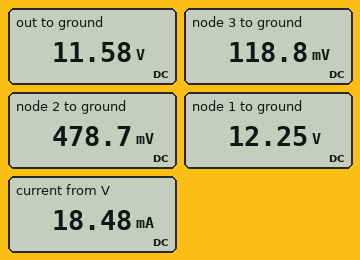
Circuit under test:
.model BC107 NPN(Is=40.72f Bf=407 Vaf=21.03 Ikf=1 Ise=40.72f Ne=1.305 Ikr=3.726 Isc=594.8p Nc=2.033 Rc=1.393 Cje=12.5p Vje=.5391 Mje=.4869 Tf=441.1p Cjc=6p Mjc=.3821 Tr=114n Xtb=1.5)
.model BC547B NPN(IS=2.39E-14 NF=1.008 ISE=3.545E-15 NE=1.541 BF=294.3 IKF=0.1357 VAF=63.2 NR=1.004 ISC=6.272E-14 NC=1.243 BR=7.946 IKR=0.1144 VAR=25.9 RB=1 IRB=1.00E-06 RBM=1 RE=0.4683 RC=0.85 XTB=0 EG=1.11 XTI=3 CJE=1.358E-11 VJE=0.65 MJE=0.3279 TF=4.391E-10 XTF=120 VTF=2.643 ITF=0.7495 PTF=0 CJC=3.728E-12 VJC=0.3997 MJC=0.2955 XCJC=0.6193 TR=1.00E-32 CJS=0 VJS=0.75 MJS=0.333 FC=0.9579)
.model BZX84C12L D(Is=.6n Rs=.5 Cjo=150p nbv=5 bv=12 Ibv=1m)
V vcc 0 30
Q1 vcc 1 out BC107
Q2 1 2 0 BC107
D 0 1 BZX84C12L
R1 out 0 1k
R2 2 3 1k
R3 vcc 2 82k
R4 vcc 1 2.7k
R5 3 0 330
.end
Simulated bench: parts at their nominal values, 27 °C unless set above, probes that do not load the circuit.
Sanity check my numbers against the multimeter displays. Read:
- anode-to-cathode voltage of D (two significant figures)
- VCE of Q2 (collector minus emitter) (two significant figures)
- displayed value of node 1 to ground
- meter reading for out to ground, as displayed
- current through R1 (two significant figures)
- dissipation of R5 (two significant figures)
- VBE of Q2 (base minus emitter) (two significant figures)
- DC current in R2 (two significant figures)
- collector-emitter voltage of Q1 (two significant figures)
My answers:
-12 V
12 V
12.25 V
11.58 V
12 mA
43 µW
480 mV
360 µA
18 V
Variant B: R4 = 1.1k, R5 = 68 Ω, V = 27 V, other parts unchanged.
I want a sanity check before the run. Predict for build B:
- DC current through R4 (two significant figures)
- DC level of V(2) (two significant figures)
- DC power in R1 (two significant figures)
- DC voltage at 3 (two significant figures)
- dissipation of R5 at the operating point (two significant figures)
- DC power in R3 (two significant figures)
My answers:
13 mA
350 mV
140 mW
22 mV
7.2 µW
8.7 mW
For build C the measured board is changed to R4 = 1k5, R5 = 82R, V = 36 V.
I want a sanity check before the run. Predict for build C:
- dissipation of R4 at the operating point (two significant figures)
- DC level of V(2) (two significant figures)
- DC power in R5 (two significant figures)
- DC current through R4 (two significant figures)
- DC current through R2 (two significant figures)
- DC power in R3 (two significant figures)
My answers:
370 mW
470 mV
15 µW
16 mA
430 µA
15 mW
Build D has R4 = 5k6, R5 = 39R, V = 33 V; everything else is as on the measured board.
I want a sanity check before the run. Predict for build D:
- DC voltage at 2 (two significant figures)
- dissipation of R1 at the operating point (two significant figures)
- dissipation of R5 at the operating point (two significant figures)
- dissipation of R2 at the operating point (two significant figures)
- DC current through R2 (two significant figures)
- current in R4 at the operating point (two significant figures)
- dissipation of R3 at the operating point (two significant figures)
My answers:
410 mV
130 mW
6.2 µW
160 µW
400 µA
3.7 mA
13 mW
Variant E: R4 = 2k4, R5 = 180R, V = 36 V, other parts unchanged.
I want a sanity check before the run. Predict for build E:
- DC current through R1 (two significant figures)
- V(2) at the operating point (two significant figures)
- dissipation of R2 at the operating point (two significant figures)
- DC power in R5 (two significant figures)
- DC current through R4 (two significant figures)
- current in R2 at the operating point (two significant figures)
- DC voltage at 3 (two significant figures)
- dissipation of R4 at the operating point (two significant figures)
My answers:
12 mA
510 mV
190 µW
34 µW
9.9 mA
430 µA
78 mV
230 mW
